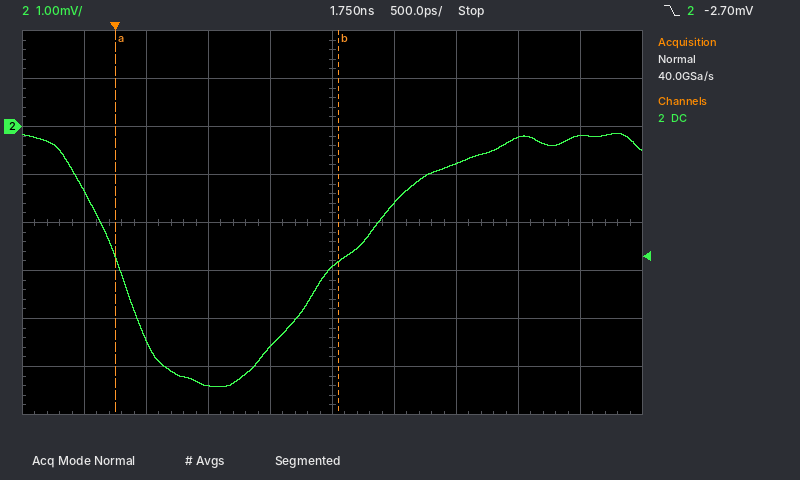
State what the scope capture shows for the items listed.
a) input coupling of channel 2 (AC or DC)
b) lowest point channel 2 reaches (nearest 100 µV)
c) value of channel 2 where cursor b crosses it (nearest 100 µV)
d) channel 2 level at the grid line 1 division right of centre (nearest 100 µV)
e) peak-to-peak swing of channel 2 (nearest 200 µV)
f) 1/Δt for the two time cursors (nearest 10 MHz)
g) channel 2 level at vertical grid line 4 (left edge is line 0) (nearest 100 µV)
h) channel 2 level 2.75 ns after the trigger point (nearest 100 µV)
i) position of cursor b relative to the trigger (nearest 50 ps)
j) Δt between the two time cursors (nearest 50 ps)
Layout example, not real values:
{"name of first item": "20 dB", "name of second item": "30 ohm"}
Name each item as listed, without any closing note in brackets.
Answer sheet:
{"input coupling of channel 2": "DC", "lowest point channel 2 reaches": "-5.4 mV", "value of channel 2 where cursor b crosses it": "-2.8 mV", "channel 2 level at the grid line 1 division right of centre": "-1.6 mV", "peak-to-peak swing of channel 2": "5.2 mV", "1/Δt for the two time cursors": "560 MHz", "channel 2 level at vertical grid line 4 (left edge is line 0)": "-4.6 mV", "channel 2 level 2.75 ns after the trigger point": "-800 µV", "position of cursor b relative to the trigger": "+1.80 ns", "Δt between the two time cursors": "1.80 ns"}
